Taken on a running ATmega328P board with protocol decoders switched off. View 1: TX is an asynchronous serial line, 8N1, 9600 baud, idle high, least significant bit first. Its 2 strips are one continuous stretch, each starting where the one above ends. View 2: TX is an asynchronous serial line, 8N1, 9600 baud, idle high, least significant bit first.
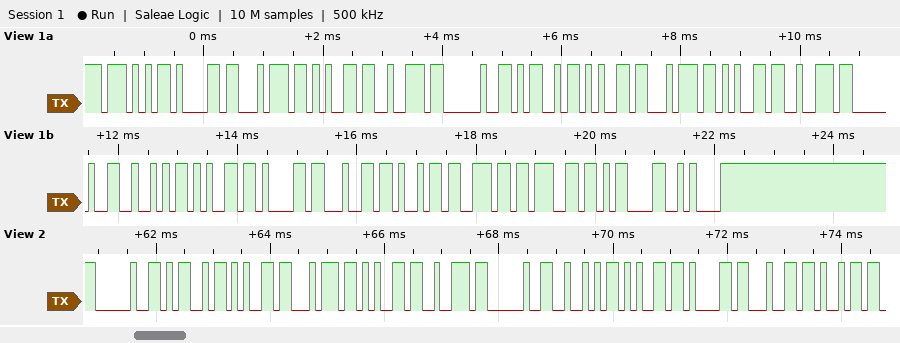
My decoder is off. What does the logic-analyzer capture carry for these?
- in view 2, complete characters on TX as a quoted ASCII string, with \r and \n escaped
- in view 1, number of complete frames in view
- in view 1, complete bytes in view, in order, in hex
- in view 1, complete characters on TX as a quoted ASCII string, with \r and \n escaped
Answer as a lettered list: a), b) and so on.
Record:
a) " Meter Readi"
b) 21
c) 57 61 74 65 72 20 4D 65 74 65 72 20 52 65 61 64 69 6E 67 0D 0A
d) "Water Meter Reading\r\n"
